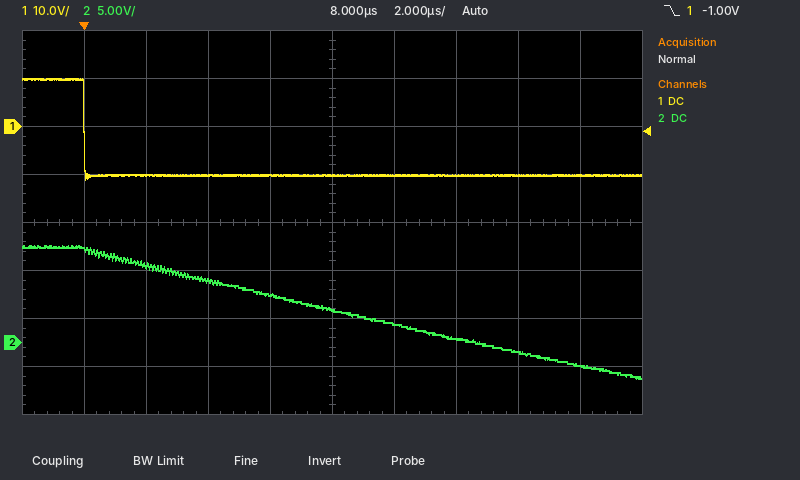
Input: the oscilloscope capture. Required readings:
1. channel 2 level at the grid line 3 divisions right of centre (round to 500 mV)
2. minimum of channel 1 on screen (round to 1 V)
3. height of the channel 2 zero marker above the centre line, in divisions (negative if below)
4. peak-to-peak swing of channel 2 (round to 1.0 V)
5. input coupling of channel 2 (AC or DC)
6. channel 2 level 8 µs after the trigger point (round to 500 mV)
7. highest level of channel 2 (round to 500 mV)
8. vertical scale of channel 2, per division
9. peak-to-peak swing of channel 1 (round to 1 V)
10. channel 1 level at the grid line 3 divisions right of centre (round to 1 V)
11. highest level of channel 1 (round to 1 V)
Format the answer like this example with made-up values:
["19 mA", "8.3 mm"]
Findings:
["-1.0 V", "-11 V", "-2.5 div", "14.0 V", "DC", "3.5 V", "10.0 V", "5 V", "21 V", "-10 V", "10 V"]
